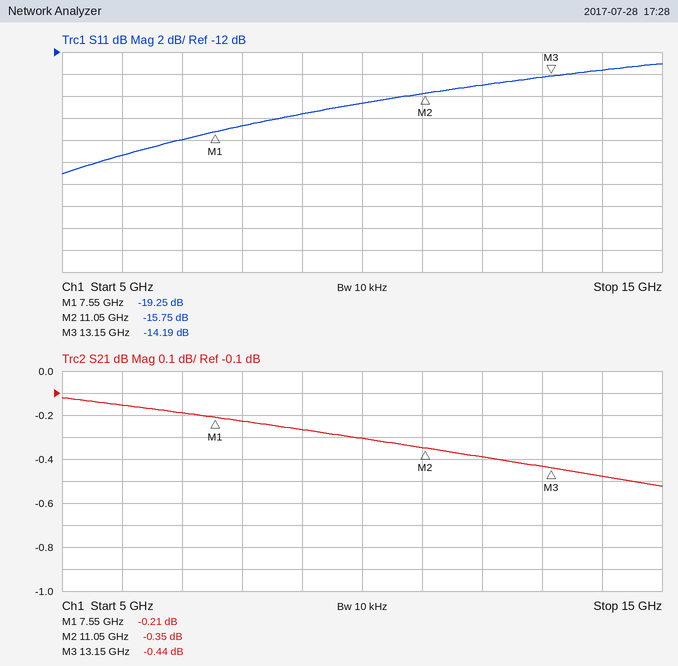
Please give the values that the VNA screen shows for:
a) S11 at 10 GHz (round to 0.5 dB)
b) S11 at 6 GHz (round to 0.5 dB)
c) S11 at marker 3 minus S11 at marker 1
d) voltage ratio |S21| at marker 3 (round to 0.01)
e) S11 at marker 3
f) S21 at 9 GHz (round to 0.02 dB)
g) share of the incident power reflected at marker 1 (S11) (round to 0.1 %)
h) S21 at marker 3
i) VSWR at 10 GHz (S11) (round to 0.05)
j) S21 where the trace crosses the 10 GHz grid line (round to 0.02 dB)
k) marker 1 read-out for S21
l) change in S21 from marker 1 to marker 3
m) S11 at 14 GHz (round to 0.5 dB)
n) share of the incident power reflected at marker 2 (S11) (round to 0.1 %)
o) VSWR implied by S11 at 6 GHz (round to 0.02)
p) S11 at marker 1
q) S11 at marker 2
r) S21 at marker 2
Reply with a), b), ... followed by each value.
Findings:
a) -16.5 dB
b) -21.5 dB
c) 5.06 dB
d) 0.95
e) -14.19 dB
f) -0.26 dB
g) 1.2 %
h) -0.44 dB
i) 1.35
j) -0.30 dB
k) -0.21 dB
l) -0.23 dB
m) -13.5 dB
n) 2.7 %
o) 1.18
p) -19.25 dB
q) -15.75 dB
r) -0.35 dB
